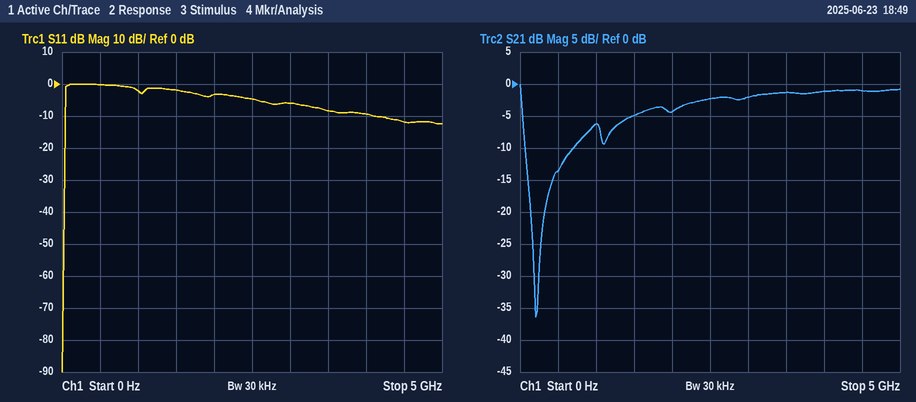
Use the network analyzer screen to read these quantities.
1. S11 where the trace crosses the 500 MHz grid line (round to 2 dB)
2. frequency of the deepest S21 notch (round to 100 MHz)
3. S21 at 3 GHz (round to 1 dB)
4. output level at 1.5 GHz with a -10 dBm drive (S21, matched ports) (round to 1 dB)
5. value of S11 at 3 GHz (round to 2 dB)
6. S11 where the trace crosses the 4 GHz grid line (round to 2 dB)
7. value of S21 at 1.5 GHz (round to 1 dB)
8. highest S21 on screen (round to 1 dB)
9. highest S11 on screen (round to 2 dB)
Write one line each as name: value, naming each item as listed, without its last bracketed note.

S11 where the trace crosses the 500 MHz grid line: 0 dB
frequency of the deepest S21 notch: 200 MHz
S21 at 3 GHz: -2 dB
output level at 1.5 GHz with a -10 dBm drive (S21, matched ports): -15 dBm
value of S11 at 3 GHz: -6 dB
S11 where the trace crosses the 4 GHz grid line: -10 dB
value of S21 at 1.5 GHz: -5 dB
highest S21 on screen: 0 dB
highest S11 on screen: 0 dB
